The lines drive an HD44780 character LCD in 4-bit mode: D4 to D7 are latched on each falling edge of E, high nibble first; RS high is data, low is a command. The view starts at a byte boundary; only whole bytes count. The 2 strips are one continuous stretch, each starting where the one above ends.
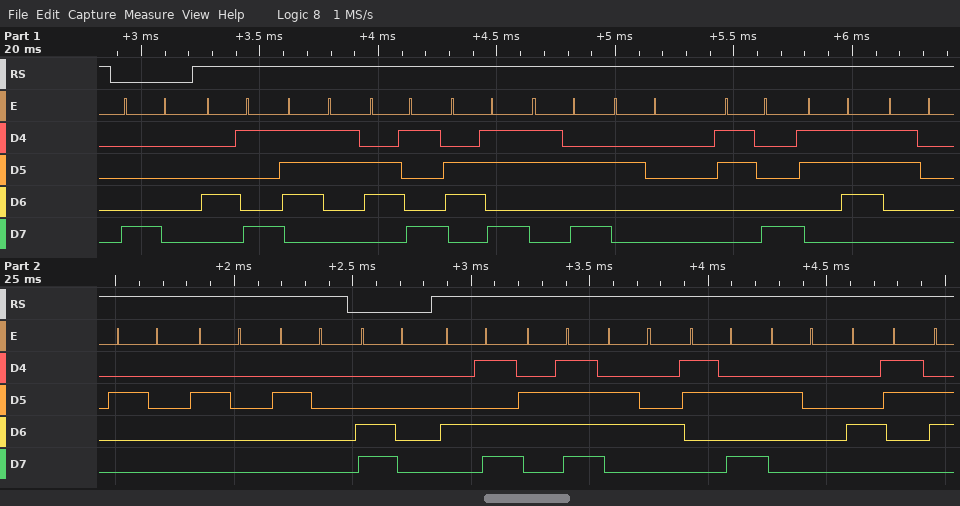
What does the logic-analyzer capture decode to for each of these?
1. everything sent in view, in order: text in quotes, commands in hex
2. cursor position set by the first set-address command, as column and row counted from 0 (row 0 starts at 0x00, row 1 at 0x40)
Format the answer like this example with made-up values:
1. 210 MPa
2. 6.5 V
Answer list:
1. 0x80 "Isik: 870   " 0xC0 "Mod: C"
2. column 0, row 0
